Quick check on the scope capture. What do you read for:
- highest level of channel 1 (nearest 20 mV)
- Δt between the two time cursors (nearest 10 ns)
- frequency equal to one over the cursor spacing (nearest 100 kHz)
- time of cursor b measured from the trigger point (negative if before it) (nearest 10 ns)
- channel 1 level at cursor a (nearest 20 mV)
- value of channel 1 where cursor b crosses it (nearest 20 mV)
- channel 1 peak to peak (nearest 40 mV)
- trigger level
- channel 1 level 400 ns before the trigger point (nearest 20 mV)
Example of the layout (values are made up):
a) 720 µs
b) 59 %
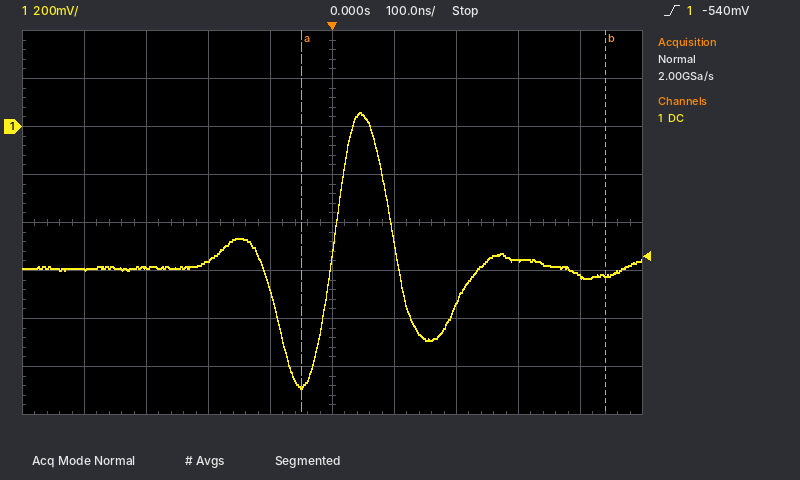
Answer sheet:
a) 60 mV
b) 490 ns
c) 2.0 MHz
d) +440 ns
e) -1.08 V
f) -620 mV
g) 1.16 V
h) -540 mV
i) -600 mV
